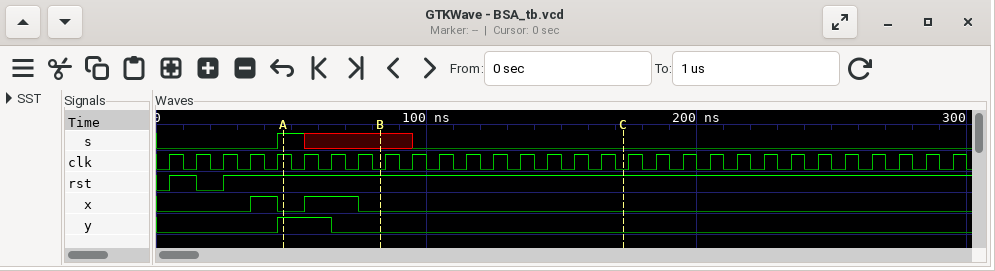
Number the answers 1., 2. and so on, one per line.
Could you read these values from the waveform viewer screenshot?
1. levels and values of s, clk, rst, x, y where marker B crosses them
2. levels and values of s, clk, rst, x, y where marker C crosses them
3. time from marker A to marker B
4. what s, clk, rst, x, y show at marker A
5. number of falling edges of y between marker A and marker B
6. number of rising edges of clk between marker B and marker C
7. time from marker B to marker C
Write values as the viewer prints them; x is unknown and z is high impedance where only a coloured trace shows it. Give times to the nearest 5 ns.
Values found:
1. s=x, clk=0, rst=1, x=0, y=0
2. s=0, clk=0, rst=1, x=0, y=0
3. 35 ns
4. s=1, clk=1, rst=1, x=0, y=1
5. 1
6. 9
7. 90 ns
